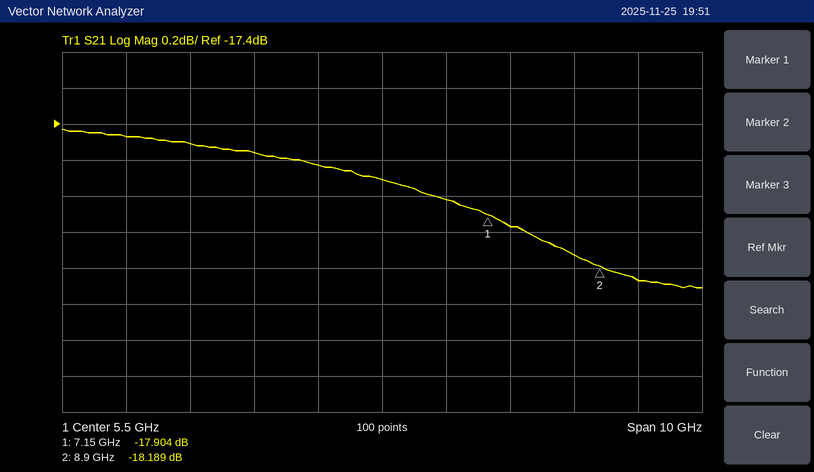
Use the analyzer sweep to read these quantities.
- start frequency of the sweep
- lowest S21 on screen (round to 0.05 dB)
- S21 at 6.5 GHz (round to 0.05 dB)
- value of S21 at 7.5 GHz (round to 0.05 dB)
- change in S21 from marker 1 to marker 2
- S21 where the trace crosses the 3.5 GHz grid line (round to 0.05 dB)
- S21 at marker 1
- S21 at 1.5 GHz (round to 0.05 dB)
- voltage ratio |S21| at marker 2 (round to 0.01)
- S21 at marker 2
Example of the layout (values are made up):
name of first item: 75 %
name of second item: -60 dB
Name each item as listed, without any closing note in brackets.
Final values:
start frequency of the sweep: 500 MHz
lowest S21 on screen: -18.30 dB
S21 at 6.5 GHz: -17.80 dB
value of S21 at 7.5 GHz: -17.95 dB
change in S21 from marker 1 to marker 2: -0.285 dB
S21 where the trace crosses the 3.5 GHz grid line: -17.55 dB
S21 at marker 1: -17.904 dB
S21 at 1.5 GHz: -17.45 dB
voltage ratio |S21| at marker 2: 0.12
S21 at marker 2: -18.189 dB
